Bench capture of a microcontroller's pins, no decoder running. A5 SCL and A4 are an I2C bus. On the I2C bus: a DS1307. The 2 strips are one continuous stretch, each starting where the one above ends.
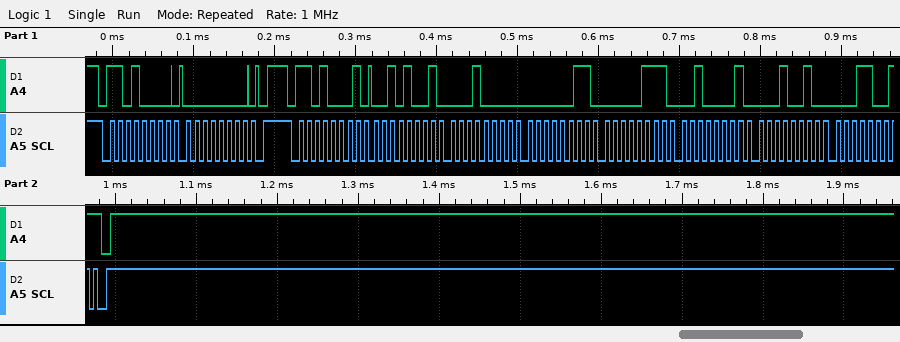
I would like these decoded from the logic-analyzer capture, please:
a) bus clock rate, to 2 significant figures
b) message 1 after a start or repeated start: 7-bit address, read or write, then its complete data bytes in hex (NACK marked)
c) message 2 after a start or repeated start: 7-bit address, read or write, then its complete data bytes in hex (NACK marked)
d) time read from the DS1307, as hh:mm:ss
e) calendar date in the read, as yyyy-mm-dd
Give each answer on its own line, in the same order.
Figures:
100 kHz
0x68 write: 00
0x68 read: 29 10 03 07 21 12 19 NACK
03:10:29
2019-12-21
